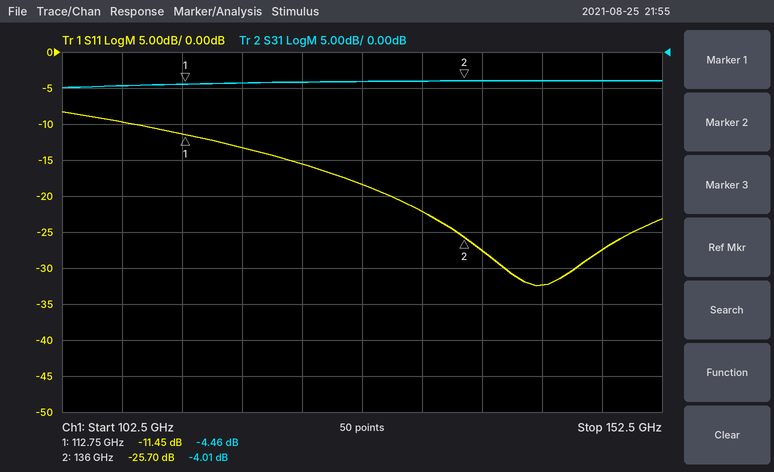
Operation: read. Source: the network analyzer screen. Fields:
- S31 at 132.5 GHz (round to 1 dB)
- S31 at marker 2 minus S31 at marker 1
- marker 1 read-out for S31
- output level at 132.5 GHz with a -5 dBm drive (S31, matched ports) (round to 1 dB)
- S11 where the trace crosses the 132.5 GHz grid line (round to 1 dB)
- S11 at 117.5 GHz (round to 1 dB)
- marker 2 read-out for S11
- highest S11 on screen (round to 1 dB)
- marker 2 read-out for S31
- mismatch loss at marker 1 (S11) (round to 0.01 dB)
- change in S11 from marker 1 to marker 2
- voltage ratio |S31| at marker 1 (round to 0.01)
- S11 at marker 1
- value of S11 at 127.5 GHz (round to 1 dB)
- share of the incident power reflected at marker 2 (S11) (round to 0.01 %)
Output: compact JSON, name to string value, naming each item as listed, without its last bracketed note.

{"S31 at 132.5 GHz": "-4 dB", "S31 at marker 2 minus S31 at marker 1": "0.45 dB", "marker 1 read-out for S31": "-4.46 dB", "output level at 132.5 GHz with a -5 dBm drive (S31, matched ports)": "-9 dBm", "S11 where the trace crosses the 132.5 GHz grid line": "-22 dB", "S11 at 117.5 GHz": "-13 dB", "marker 2 read-out for S11": "-25.70 dB", "highest S11 on screen": "-8 dB", "marker 2 read-out for S31": "-4.01 dB", "mismatch loss at marker 1 (S11)": "0.32 dB", "change in S11 from marker 1 to marker 2": "-14.25 dB", "voltage ratio |S31| at marker 1": "0.60", "S11 at marker 1": "-11.45 dB", "value of S11 at 127.5 GHz": "-18 dB", "share of the incident power reflected at marker 2 (S11)": "0.27 %"}
